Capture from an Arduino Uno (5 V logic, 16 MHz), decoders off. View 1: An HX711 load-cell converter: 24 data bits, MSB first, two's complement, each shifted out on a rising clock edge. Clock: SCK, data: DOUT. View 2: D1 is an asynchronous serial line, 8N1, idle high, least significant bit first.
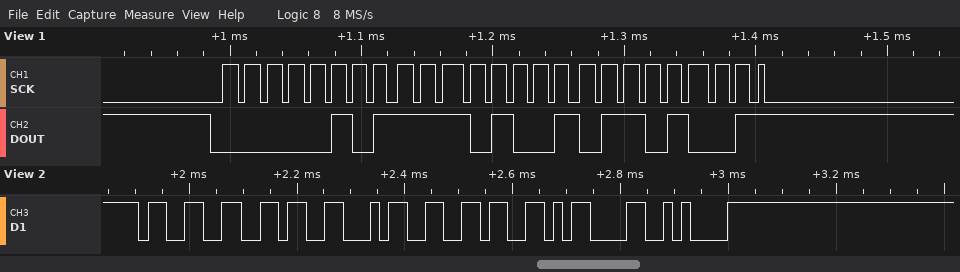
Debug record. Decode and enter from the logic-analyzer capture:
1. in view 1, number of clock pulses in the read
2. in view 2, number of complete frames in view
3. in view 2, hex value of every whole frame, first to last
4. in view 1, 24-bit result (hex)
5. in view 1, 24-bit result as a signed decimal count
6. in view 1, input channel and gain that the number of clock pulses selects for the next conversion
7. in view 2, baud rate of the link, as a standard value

25
6
0x33 0x36 0x34 0x36 0x0D 0x0A
0x05E969
387433
channel A, gain 128
57600 baud
